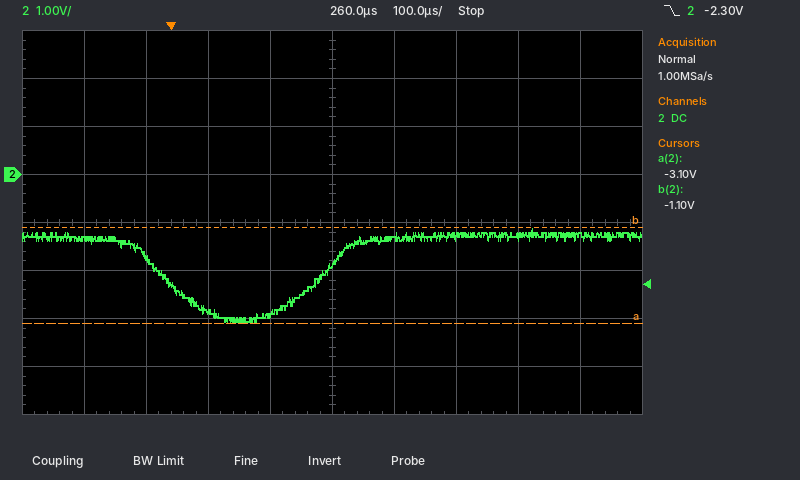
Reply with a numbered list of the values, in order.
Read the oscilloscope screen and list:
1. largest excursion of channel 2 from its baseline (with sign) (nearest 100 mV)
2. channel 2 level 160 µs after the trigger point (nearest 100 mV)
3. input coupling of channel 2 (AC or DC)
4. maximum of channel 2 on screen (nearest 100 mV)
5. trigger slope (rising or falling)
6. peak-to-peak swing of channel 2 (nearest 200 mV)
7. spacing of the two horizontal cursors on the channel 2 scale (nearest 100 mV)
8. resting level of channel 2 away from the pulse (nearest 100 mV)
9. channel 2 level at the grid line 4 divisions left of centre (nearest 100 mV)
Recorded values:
1. -1.8 V
2. -2.9 V
3. DC
4. -1.1 V
5. falling
6. 2.0 V
7. 2.0 V
8. -1.3 V
9. -1.3 V
